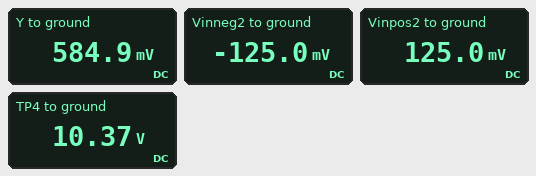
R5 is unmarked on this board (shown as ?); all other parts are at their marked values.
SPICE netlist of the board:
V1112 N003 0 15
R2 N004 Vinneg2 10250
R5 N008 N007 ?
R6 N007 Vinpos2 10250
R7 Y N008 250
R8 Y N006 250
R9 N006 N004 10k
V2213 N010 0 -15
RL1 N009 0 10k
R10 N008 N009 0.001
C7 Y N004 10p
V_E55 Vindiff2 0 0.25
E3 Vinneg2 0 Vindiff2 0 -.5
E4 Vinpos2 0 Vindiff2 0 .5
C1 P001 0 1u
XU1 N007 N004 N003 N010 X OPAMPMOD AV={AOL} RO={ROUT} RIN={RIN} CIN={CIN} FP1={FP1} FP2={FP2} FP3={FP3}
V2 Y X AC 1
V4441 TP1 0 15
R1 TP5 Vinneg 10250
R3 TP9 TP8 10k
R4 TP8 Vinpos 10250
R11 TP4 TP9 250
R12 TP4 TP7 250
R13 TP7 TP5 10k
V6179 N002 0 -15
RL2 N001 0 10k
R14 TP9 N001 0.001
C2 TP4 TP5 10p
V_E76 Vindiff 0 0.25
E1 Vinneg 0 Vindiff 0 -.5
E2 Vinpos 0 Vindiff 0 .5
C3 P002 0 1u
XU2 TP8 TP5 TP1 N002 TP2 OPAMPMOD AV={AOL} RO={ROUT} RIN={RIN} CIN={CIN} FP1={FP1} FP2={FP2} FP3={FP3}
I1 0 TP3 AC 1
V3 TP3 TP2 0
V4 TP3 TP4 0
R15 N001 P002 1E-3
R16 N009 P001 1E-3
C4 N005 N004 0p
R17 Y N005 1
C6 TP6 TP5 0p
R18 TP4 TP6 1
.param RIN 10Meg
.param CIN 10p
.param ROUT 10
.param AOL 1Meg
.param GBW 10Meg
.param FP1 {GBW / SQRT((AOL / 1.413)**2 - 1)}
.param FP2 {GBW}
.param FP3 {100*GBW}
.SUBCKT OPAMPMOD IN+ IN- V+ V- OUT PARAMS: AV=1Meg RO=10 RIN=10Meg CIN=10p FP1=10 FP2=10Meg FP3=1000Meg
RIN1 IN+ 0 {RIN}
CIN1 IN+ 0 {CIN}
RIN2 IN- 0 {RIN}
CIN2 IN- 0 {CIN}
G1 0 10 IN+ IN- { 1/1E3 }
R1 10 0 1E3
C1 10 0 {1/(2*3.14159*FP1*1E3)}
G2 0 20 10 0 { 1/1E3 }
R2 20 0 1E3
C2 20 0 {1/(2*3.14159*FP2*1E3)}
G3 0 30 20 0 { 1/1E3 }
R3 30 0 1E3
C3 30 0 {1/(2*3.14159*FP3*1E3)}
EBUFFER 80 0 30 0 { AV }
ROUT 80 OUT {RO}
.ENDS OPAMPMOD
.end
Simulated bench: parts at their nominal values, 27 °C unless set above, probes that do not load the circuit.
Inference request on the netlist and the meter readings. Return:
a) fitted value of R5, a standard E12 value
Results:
33 kΩ
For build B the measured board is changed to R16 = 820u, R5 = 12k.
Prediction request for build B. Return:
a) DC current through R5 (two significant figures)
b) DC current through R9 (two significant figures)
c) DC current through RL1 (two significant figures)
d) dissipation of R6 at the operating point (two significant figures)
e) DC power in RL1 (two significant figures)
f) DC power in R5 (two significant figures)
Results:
97 µA
120 µA
230 µA
95 µW
520 µW
110 µW
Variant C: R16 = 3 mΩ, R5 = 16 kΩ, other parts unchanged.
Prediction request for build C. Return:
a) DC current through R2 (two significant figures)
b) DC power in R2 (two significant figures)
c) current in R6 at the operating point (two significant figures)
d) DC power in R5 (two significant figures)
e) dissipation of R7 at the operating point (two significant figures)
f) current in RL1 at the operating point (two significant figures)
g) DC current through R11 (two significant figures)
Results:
61 µA
39 µW
37 µA
22 µW
5.4 µW
110 µA
1.5 mA
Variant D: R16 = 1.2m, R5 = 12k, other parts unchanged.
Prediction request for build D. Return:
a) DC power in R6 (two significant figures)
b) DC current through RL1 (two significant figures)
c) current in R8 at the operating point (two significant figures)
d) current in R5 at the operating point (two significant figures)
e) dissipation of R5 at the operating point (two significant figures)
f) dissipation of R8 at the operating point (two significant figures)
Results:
95 µW
230 µA
120 µA
97 µA
110 µW
3.7 µW
